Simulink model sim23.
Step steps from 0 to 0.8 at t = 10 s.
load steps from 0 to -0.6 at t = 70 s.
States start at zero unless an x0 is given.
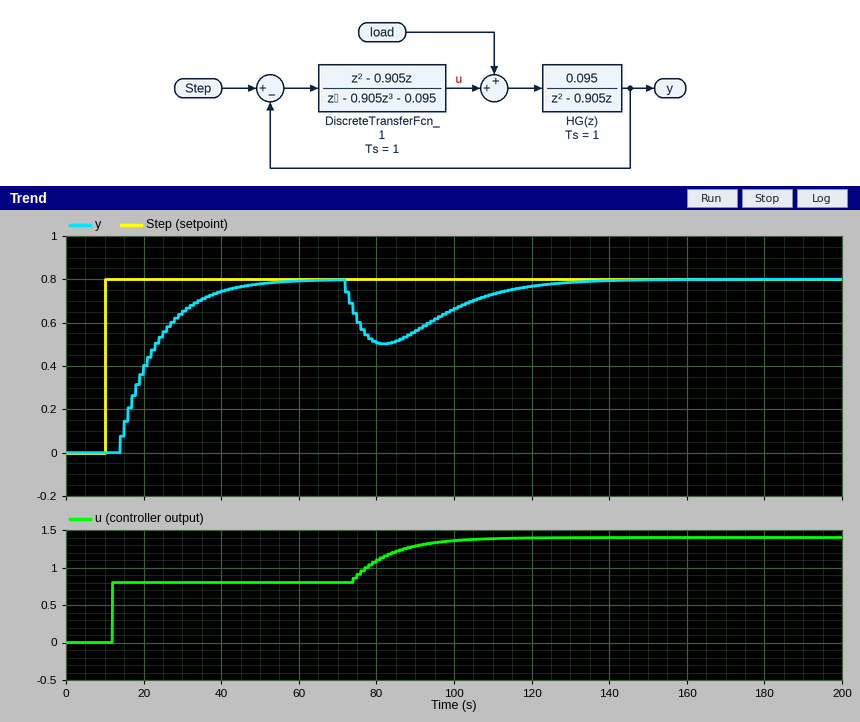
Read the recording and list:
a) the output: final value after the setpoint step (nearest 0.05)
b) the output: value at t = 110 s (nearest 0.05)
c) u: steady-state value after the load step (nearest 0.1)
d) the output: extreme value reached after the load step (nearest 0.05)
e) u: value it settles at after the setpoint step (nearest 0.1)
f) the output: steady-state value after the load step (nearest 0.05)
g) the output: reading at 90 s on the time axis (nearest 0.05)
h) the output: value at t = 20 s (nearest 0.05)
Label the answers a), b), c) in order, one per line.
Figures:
a) 0.80
b) 0.75
c) 1.4
d) 0.50
e) 0.8
f) 0.80
g) 0.55
h) 0.40
